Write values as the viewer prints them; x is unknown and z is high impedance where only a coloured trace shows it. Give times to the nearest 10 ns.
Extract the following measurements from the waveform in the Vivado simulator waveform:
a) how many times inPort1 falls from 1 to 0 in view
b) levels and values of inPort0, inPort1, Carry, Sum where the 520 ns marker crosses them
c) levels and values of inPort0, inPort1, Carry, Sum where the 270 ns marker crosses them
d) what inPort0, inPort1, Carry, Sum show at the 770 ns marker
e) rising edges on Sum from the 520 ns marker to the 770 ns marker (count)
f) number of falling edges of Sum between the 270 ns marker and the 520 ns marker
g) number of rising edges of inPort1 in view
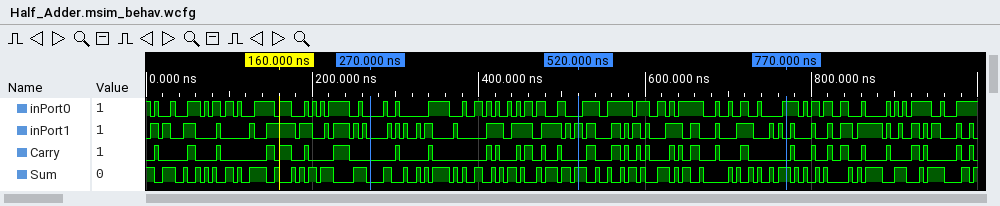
45
inPort0=0, inPort1=1, Carry=0, Sum=1
inPort0=0, inPort1=0, Carry=0, Sum=0
inPort0=1, inPort1=0, Carry=0, Sum=1
15
15
45
